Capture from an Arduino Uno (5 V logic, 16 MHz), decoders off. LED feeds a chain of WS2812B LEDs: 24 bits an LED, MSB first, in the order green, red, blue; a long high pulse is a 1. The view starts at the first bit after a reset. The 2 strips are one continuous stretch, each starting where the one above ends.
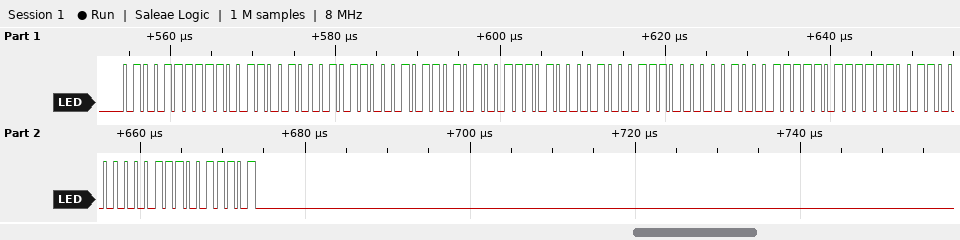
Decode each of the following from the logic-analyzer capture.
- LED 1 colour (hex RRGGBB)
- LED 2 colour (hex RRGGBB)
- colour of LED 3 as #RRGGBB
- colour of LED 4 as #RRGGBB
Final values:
#CC4F8B
#A71642
#1138F7
#03E69D
